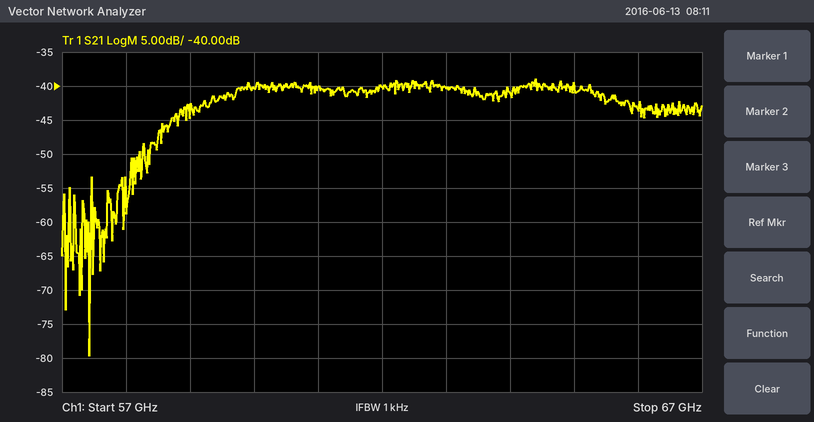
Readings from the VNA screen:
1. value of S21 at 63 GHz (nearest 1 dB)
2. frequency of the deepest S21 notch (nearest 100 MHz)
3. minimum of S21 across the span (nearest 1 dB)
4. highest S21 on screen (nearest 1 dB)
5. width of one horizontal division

-40 dB
57.4 GHz
-80 dB
-39 dB
1 GHz
